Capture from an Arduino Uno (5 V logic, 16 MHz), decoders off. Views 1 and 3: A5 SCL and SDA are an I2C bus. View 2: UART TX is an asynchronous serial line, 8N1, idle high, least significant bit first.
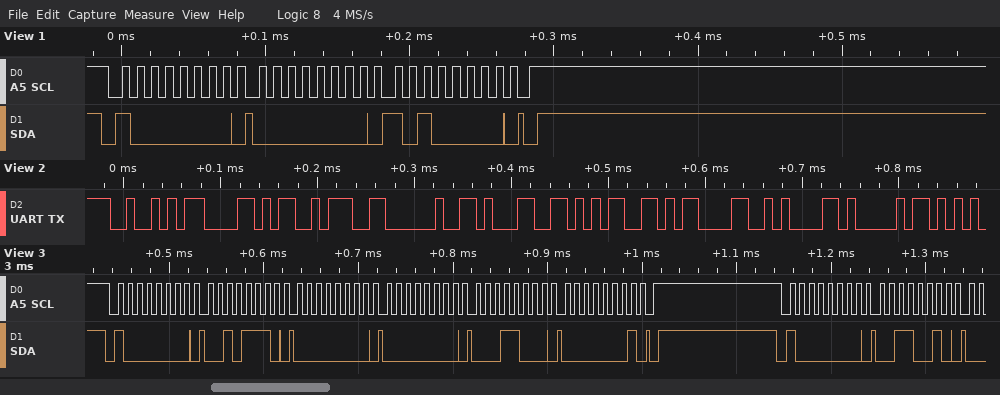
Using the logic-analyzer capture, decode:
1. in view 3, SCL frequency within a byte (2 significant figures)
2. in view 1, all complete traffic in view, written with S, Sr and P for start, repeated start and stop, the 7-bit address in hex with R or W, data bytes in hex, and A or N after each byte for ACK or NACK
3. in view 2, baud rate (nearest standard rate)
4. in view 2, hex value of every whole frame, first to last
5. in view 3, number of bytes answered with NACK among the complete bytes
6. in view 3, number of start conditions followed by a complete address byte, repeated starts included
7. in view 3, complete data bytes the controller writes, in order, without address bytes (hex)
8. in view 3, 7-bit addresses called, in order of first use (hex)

100 kHz
S 40W A 00 A A0 A P
115200 baud
52 58 3A 20 31 35 0D 0A 41
0
2
2E 00 00 18 01 32
0x40
